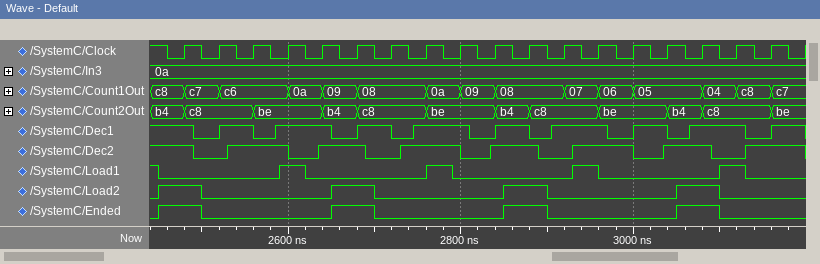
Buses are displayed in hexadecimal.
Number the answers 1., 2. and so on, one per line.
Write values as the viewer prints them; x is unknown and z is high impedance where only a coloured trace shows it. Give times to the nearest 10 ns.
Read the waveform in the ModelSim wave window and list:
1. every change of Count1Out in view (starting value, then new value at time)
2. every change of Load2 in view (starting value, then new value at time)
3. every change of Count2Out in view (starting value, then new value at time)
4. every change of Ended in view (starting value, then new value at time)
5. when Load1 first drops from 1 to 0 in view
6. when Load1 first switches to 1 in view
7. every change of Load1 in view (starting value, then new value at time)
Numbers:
1. c8, c7 at 2480 ns, c6 at 2520 ns, 0a at 2600 ns, 09 at 2640 ns, 08 at 2680 ns, 0a at 2760 ns, 09 at 2800 ns, 08 at 2840 ns, 07 at 2920 ns, 06 at 2960 ns, 05 at 3000 ns, 04 at 3080 ns, c8 at 3120 ns, c7 at 3160 ns
2. 0, 1 at 2450 ns, 0 at 2500 ns, 1 at 2650 ns, 0 at 2700 ns, 1 at 2850 ns, 0 at 2900 ns, 1 at 3050 ns, 0 at 3100 ns
3. b4, c8 at 2480 ns, be at 2560 ns, b4 at 2640 ns, c8 at 2680 ns, be at 2760 ns, b4 at 2840 ns, c8 at 2880 ns, be at 2960 ns, b4 at 3040 ns, c8 at 3080 ns, be at 3160 ns
4. 0, 1 at 2450 ns, 0 at 2500 ns, 1 at 2650 ns, 0 at 2700 ns, 1 at 2850 ns, 0 at 2900 ns, 1 at 3050 ns, 0 at 3100 ns
5. 2450 ns
6. 2590 ns
7. 1, 0 at 2450 ns, 1 at 2590 ns, 0 at 2620 ns, 1 at 2760 ns, 0 at 2790 ns, 1 at 2930 ns, 0 at 2960 ns, 1 at 3100 ns, 0 at 3130 ns
